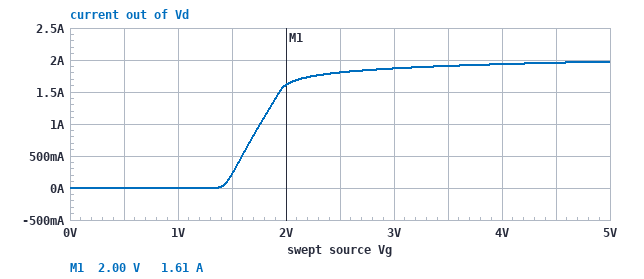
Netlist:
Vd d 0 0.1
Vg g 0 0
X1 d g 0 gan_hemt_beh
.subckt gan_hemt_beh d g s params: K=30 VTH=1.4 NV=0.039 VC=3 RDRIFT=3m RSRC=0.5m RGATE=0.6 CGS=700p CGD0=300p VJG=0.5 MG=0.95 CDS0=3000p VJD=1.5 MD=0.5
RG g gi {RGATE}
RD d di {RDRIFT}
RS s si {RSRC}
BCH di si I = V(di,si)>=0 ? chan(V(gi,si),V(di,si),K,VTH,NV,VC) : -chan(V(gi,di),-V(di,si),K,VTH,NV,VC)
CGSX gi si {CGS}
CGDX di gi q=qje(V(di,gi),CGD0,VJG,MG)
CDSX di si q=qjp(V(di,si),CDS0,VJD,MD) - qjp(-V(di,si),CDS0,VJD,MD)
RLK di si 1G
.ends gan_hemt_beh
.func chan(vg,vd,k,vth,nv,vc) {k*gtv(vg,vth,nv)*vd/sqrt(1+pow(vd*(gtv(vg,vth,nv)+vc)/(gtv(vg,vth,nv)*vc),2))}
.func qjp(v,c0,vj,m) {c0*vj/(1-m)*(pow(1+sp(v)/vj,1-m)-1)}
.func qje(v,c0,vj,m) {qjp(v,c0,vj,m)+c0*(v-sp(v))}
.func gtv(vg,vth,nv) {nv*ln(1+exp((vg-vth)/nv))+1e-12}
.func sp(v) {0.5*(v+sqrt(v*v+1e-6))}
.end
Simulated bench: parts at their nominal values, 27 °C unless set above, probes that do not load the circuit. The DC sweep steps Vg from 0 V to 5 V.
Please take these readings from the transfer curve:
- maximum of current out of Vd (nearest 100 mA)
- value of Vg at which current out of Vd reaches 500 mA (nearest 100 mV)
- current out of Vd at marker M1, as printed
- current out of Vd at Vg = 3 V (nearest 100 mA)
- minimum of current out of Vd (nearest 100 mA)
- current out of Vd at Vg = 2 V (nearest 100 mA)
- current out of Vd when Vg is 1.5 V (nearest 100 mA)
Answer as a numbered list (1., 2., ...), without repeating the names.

1. 2.0 A
2. 1.6 V
3. 1.61 A
4. 1.9 A
5. 0 A
6. 1.6 A
7. 200 mA
